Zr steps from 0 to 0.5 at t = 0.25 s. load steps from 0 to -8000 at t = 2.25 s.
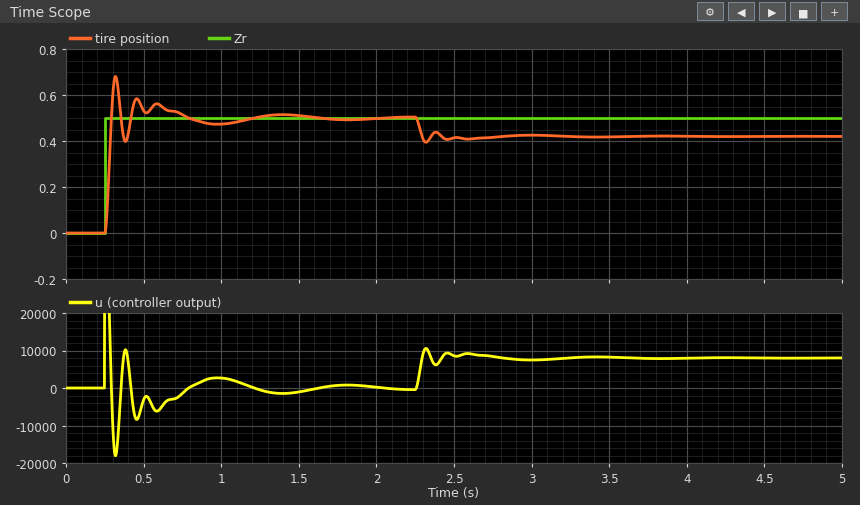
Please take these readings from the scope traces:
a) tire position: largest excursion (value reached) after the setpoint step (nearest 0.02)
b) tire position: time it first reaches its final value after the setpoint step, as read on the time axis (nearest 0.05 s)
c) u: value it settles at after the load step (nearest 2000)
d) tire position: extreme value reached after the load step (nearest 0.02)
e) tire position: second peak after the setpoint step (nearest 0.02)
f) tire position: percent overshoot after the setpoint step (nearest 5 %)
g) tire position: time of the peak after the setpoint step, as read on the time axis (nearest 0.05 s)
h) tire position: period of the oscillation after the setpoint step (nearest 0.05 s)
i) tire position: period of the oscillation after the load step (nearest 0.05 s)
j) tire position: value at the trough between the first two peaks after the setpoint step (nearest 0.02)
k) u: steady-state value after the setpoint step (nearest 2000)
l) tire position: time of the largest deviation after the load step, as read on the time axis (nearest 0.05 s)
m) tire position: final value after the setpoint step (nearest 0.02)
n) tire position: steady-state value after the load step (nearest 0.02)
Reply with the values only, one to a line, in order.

0.68
0.30 s
8000
0.40
0.58
35 %
0.30 s
0.15 s
0.15 s
0.40
0
2.30 s
0.50
0.42
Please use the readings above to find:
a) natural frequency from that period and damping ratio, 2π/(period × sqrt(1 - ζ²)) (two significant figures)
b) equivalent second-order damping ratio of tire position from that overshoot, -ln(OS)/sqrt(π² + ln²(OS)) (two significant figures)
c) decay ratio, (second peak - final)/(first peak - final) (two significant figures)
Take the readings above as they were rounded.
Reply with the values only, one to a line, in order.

44 rad/s
0.32
0.44
